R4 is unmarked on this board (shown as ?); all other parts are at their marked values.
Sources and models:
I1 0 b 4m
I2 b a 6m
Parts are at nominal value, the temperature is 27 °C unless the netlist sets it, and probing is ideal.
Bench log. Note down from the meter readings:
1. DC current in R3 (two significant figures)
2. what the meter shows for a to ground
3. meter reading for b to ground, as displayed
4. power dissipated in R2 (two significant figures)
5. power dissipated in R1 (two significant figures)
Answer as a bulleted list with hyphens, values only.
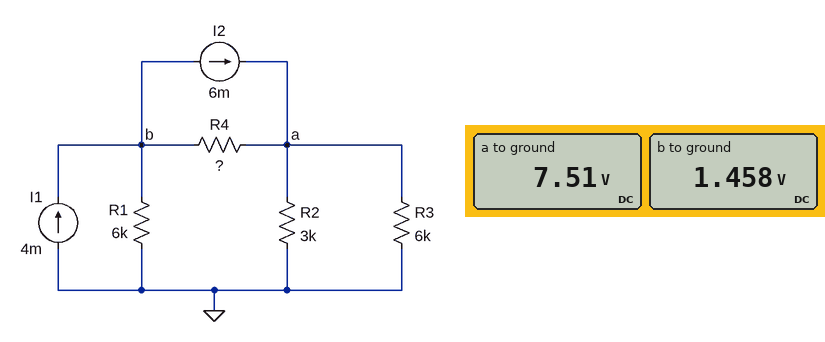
- 1.3 mA
- 7.51 V
- 1.458 V
- 19 mW
- 350 µW
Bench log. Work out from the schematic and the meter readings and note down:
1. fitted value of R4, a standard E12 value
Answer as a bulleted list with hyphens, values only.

- 2.7 kΩ
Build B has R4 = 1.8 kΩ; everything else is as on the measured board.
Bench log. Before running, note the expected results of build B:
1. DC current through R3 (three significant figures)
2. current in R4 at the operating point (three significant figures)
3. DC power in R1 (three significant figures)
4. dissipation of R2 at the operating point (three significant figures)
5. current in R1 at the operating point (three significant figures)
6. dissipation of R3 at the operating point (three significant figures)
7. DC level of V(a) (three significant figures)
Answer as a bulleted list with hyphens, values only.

- 1.18 mA
- 2.45 mA
- 1.21 mW
- 16.8 mW
- 449 µA
- 8.41 mW
- 7.10 V
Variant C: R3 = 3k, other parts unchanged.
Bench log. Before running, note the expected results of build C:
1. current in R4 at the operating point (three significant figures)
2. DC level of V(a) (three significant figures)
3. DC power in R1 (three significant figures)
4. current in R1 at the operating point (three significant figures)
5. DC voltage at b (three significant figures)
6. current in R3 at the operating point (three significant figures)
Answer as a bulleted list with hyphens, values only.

- 2.06 mA
- 5.91 V
- 20.8 µW
- 58.8 µA
- 353 mV
- 1.97 mA
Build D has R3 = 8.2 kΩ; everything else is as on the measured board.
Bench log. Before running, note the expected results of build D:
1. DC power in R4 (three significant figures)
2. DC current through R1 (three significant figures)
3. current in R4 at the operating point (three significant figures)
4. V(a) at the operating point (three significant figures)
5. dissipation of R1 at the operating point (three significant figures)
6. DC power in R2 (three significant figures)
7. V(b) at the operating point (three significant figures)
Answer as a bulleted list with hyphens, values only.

- 14.4 mW
- 311 µA
- 2.31 mA
- 8.10 V
- 579 µW
- 21.9 mW
- 1.86 V
